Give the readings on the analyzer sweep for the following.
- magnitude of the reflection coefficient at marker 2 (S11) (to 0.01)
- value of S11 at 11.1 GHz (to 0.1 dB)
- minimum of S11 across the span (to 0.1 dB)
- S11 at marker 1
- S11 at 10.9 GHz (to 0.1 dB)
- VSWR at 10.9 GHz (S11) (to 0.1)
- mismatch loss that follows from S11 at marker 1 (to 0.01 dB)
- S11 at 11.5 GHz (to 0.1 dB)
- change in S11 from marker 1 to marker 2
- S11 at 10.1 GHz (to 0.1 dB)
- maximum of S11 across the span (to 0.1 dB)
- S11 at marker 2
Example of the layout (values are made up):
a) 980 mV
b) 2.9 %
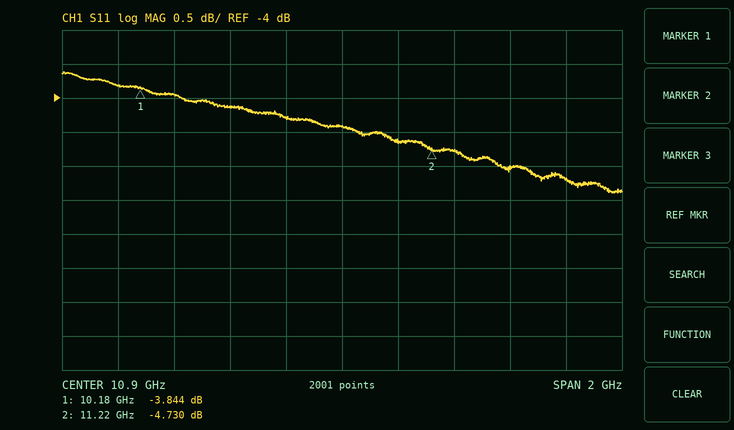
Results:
a) 0.58
b) -4.6 dB
c) -5.4 dB
d) -3.844 dB
e) -4.4 dB
f) 4.0
g) 2.31 dB
h) -5.0 dB
i) -0.886 dB
j) -3.8 dB
k) -3.6 dB
l) -4.730 dB
